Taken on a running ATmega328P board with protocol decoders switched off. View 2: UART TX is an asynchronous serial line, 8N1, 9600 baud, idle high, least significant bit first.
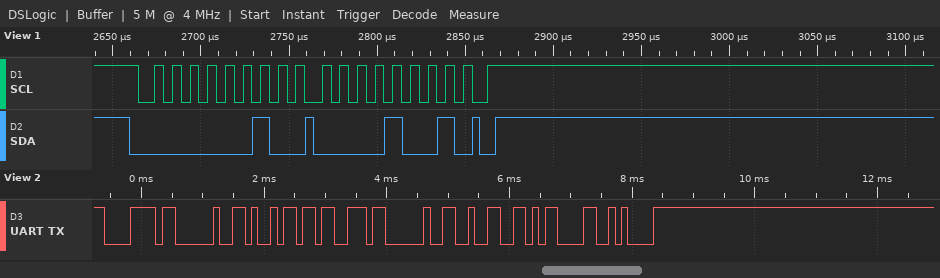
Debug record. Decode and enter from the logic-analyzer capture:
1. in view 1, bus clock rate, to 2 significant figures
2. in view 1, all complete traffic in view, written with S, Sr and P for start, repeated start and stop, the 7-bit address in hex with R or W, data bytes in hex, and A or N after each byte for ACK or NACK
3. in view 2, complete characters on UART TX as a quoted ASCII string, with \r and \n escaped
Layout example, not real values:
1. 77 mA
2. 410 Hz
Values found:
1. 100 kHz
2. S 01W A 09 A P
3. "x is 2\r\n"
